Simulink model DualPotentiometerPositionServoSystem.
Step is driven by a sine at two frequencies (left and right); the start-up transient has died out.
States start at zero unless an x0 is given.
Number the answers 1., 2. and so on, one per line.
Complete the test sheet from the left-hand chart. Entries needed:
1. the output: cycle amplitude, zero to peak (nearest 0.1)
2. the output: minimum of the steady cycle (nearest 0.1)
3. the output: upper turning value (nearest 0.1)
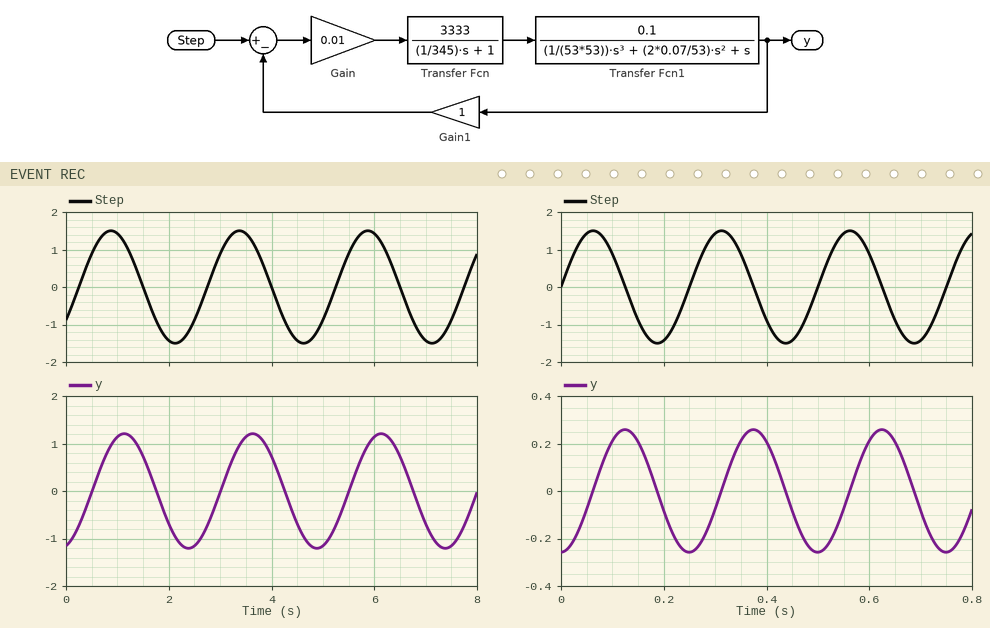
1. 1.2
2. -1.2
3. 1.2
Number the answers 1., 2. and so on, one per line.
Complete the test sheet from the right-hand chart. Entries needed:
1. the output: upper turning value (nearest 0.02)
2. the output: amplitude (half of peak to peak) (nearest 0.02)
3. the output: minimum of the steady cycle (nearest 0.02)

1. 0.26
2. 0.26
3. -0.26
